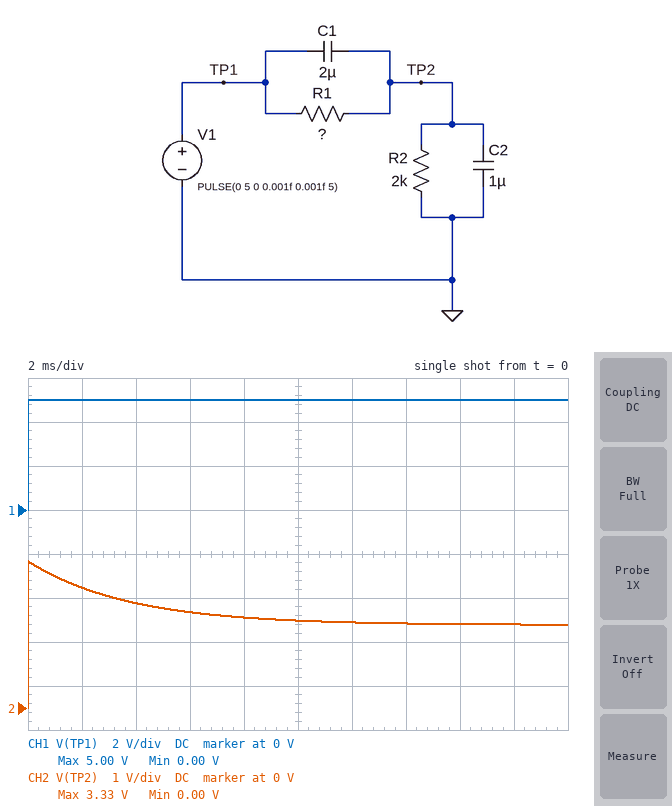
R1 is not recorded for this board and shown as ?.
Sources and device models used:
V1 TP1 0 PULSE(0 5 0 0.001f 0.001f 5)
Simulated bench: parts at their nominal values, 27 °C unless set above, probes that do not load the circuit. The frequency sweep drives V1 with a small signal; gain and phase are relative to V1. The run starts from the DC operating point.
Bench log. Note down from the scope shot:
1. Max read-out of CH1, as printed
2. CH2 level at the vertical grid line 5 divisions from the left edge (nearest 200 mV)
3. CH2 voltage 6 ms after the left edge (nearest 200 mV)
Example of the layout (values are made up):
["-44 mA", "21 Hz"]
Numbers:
["5.00 V", "2.0 V", "2.2 V"]
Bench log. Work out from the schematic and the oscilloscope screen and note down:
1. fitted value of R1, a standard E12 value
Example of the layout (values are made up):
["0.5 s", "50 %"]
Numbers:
["3.3 kΩ"]
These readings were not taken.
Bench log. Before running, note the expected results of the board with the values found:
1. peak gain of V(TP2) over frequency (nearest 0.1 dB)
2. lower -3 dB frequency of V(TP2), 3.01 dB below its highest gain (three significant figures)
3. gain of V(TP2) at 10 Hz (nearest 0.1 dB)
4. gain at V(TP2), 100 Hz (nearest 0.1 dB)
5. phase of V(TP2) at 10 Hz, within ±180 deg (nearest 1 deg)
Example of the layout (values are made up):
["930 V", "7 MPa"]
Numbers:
["-3.5 dB", "25.5 Hz", "-8.0 dB", "-4.0 dB", "9 deg"]
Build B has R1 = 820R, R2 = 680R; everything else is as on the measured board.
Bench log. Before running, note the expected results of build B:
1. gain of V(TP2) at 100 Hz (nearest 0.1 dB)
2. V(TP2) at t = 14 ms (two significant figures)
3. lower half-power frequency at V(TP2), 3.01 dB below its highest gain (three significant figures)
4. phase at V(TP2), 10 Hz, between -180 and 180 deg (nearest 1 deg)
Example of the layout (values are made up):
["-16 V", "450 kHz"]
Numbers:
["-5.5 dB", "2.3 V", "39.1 Hz", "2 deg"]
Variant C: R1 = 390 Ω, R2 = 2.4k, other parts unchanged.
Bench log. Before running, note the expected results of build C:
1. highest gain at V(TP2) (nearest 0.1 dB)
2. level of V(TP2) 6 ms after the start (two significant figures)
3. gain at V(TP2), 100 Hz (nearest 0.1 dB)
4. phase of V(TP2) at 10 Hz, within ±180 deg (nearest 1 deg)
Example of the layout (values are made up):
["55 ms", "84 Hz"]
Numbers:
["-1.3 dB", "4.3 V", "-1.8 dB", "-1 deg"]
